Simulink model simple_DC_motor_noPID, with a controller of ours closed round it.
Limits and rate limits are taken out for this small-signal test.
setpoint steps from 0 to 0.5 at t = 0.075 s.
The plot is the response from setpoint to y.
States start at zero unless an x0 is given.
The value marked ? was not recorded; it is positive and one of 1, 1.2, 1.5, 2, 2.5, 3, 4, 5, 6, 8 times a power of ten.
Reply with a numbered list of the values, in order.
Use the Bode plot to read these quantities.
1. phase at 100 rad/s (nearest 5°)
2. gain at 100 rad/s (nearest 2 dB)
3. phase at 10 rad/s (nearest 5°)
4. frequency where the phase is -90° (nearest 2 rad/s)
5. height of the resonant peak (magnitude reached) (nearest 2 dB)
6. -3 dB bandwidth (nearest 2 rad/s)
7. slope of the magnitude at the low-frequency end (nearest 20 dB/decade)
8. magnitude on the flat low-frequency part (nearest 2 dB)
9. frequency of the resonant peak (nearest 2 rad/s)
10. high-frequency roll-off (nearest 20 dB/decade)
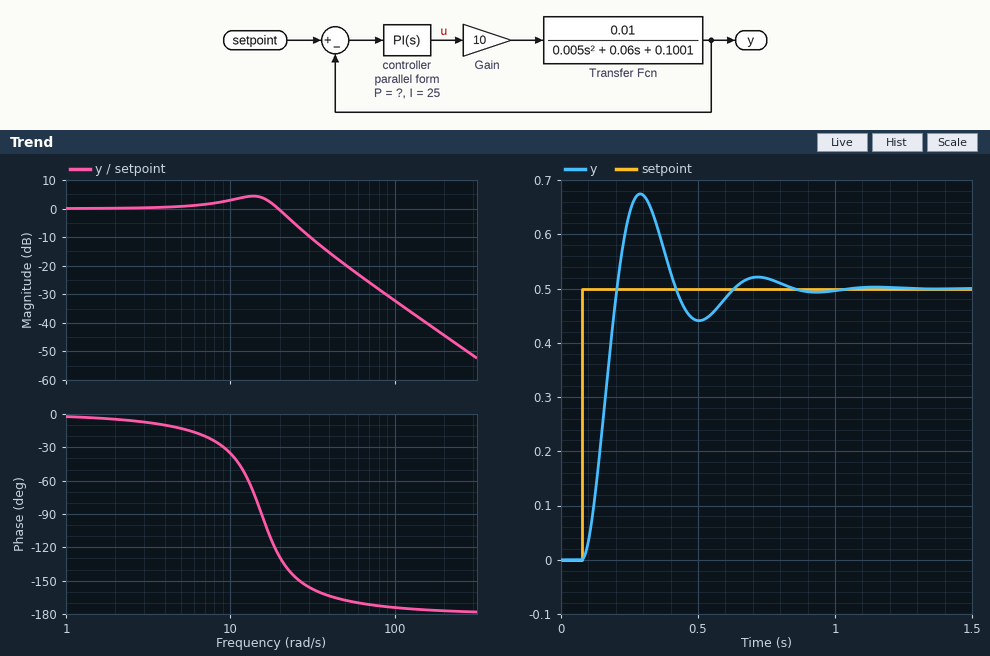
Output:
1. -175°
2. -32 dB
3. -35°
4. 16 rad/s
5. 4 dB
6. 22 rad/s
7. 0 dB/decade
8. 0 dB
9. 14 rad/s
10. -40 dB/decade
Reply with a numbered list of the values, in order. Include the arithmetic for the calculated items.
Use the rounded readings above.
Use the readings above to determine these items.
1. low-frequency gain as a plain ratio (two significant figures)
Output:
1. 10^(0 / 20) = 1.0
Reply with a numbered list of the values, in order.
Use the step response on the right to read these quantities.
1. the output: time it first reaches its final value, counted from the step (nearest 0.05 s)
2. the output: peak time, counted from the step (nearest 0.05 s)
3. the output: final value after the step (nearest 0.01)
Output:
1. 0.15 s
2. 0.20 s
3. 0.50
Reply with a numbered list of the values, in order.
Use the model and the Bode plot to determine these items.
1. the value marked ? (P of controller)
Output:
1. 12
